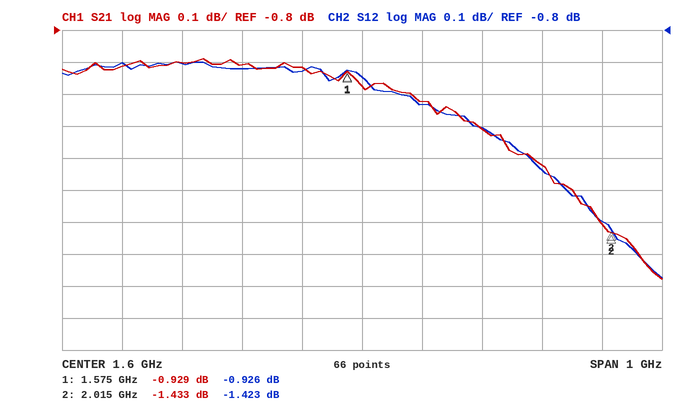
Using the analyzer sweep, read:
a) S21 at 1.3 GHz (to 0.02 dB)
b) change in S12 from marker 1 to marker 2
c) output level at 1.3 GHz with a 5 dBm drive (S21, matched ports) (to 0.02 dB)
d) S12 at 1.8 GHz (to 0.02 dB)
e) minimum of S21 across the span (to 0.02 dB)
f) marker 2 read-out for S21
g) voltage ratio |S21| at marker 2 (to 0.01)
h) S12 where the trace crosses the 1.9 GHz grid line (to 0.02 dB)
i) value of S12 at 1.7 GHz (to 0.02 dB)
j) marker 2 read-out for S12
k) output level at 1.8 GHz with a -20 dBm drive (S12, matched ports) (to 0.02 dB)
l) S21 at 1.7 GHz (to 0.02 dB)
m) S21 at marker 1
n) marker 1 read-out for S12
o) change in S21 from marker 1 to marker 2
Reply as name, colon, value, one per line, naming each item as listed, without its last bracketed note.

S21 at 1.3 GHz: -0.90 dB
change in S12 from marker 1 to marker 2: -0.497 dB
output level at 1.3 GHz with a 5 dBm drive (S21, matched ports): 4.10 dBm
S12 at 1.8 GHz: -1.10 dB
minimum of S21 across the span: -1.58 dB
marker 2 read-out for S21: -1.433 dB
voltage ratio |S21| at marker 2: 0.85
S12 where the trace crosses the 1.9 GHz grid line: -1.24 dB
value of S12 at 1.7 GHz: -1.04 dB
marker 2 read-out for S12: -1.423 dB
output level at 1.8 GHz with a -20 dBm drive (S12, matched ports): -21.10 dBm
S21 at 1.7 GHz: -1.02 dB
S21 at marker 1: -0.929 dB
marker 1 read-out for S12: -0.926 dB
change in S21 from marker 1 to marker 2: -0.504 dB
